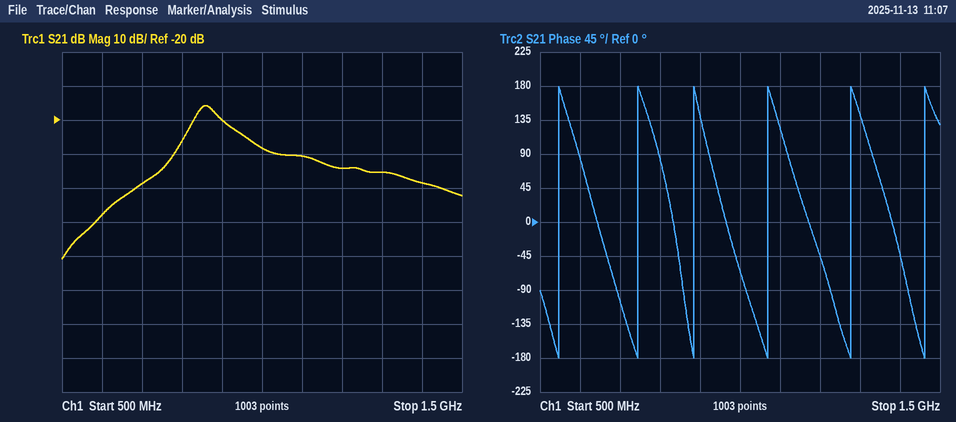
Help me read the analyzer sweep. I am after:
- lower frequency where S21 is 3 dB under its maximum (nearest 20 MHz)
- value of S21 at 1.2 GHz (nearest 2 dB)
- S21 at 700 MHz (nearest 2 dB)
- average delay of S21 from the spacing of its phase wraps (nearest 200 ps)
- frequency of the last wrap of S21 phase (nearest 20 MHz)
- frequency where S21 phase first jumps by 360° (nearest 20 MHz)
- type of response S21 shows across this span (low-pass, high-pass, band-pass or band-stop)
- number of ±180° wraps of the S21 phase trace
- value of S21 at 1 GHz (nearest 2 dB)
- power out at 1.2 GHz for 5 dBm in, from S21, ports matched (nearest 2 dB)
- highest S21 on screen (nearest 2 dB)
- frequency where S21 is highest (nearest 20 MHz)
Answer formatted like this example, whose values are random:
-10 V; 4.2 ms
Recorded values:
840 MHz; -34 dB; -38 dB; 5.4 ns; 1.46 GHz; 540 MHz; band-pass; 6; -28 dB; -30 dBm; -16 dB; 860 MHz
